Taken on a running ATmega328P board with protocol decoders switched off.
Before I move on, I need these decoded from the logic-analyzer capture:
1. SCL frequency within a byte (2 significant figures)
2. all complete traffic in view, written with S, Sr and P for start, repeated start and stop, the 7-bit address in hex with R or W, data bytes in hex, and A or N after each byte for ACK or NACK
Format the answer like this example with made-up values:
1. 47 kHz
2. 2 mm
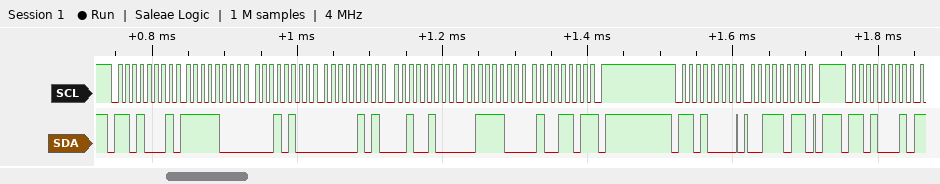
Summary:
1. 100 kHz
2. S 68R A F8 A 14 A 05 A 24 A 3C A 4D N P S 68W A 3B A P S 68R A
